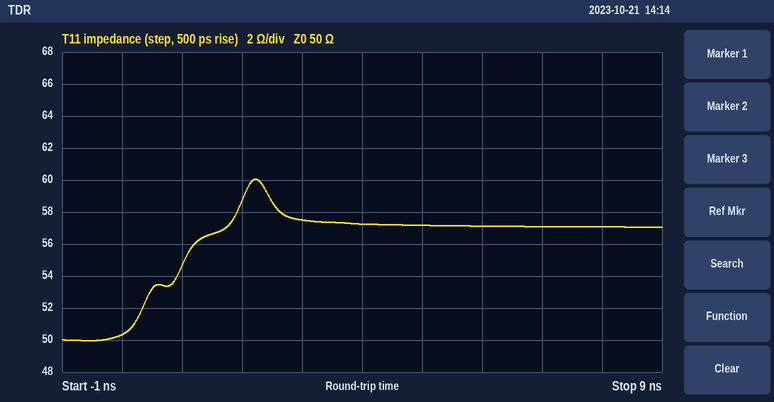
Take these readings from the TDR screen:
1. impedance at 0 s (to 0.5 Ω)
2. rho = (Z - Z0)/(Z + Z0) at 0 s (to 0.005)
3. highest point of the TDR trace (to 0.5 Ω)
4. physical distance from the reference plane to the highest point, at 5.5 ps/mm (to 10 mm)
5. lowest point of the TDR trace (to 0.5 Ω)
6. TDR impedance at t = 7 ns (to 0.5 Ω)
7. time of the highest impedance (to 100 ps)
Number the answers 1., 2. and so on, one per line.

1. 50.5 Ω
2. +0.005
3. 60.0 Ω
4. 200 mm
5. 50.0 Ω
6. 57.0 Ω
7. 2.2 ns
